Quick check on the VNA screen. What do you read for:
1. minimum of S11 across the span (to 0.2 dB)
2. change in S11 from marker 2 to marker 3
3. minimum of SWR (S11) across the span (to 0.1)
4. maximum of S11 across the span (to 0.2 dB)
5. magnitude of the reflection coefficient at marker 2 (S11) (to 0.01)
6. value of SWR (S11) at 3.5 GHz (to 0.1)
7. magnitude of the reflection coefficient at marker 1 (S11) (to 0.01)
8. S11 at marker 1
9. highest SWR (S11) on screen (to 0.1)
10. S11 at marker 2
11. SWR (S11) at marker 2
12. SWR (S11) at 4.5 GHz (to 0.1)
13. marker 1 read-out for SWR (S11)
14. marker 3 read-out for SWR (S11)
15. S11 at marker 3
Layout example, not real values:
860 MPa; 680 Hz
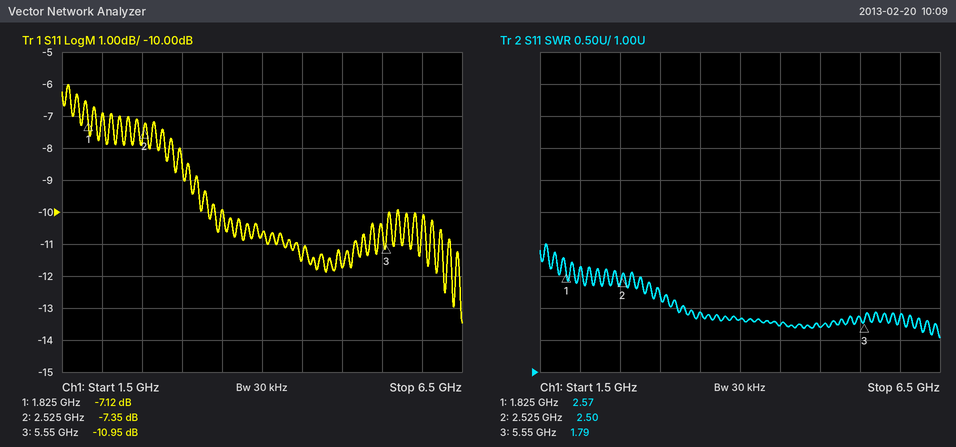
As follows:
-13.4 dB; -3.60 dB; 1.5; -6.0 dB; 0.43; 1.9; 0.44; -7.12 dB; 3.0; -7.35 dB; 2.50; 1.7; 2.57; 1.79; -10.95 dB
